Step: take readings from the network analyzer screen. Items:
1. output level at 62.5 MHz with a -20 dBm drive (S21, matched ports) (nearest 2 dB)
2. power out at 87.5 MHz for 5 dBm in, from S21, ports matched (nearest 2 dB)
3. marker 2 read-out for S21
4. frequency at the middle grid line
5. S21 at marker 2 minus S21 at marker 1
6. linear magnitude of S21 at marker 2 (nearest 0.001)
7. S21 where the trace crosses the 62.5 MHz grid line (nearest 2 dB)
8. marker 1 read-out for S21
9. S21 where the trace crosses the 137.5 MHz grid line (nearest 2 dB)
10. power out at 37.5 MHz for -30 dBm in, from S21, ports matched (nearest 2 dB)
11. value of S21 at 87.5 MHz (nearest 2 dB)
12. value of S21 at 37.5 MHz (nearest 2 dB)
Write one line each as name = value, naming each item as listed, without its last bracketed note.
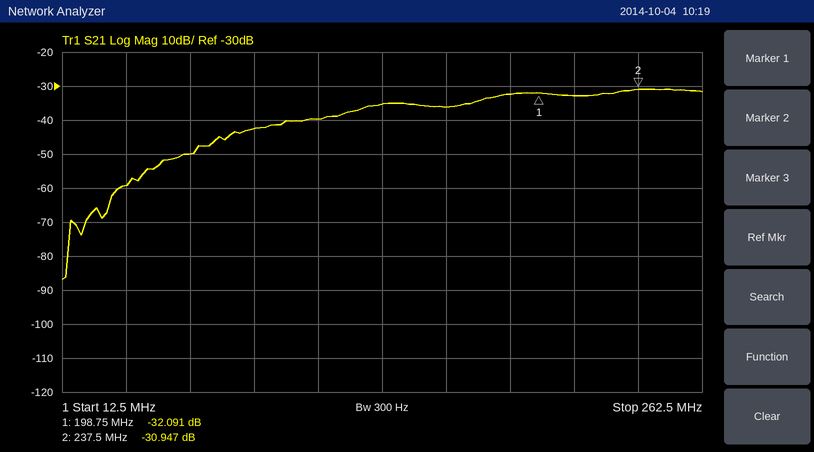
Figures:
output level at 62.5 MHz with a -20 dBm drive (S21, matched ports) = -70 dBm
power out at 87.5 MHz for 5 dBm in, from S21, ports matched = -38 dBm
marker 2 read-out for S21 = -30.947 dB
frequency at the middle grid line = 137.5 MHz
S21 at marker 2 minus S21 at marker 1 = 1.144 dB
linear magnitude of S21 at marker 2 = 0.028
S21 where the trace crosses the 62.5 MHz grid line = -50 dB
marker 1 read-out for S21 = -32.091 dB
S21 where the trace crosses the 137.5 MHz grid line = -36 dB
power out at 37.5 MHz for -30 dBm in, from S21, ports matched = -90 dBm
value of S21 at 87.5 MHz = -42 dB
value of S21 at 37.5 MHz = -60 dB
